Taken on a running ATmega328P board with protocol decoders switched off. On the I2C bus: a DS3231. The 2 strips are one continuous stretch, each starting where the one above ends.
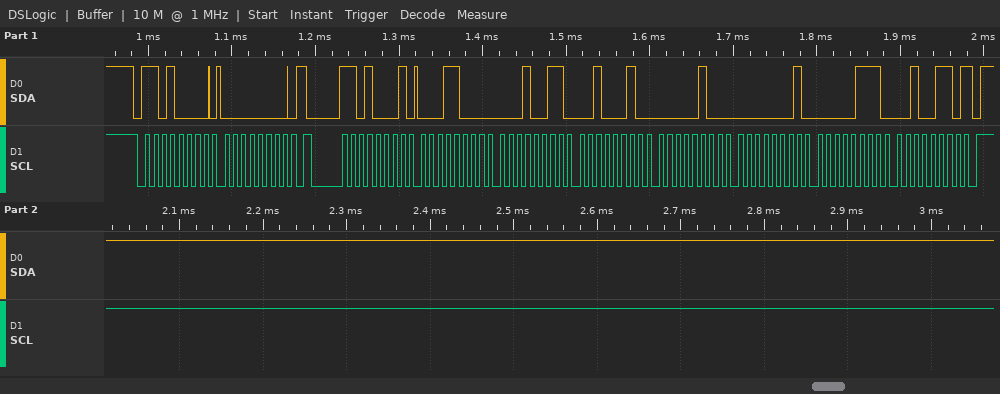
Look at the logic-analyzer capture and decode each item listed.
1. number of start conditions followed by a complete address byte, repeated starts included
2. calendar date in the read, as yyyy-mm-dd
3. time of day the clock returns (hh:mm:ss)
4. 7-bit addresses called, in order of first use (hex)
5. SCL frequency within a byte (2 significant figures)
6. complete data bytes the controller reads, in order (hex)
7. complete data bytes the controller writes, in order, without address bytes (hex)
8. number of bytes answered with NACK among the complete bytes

2
2026-07-01
22:13:18
0x68
100 kHz
18 13 22 04 01 07 26
00
1
